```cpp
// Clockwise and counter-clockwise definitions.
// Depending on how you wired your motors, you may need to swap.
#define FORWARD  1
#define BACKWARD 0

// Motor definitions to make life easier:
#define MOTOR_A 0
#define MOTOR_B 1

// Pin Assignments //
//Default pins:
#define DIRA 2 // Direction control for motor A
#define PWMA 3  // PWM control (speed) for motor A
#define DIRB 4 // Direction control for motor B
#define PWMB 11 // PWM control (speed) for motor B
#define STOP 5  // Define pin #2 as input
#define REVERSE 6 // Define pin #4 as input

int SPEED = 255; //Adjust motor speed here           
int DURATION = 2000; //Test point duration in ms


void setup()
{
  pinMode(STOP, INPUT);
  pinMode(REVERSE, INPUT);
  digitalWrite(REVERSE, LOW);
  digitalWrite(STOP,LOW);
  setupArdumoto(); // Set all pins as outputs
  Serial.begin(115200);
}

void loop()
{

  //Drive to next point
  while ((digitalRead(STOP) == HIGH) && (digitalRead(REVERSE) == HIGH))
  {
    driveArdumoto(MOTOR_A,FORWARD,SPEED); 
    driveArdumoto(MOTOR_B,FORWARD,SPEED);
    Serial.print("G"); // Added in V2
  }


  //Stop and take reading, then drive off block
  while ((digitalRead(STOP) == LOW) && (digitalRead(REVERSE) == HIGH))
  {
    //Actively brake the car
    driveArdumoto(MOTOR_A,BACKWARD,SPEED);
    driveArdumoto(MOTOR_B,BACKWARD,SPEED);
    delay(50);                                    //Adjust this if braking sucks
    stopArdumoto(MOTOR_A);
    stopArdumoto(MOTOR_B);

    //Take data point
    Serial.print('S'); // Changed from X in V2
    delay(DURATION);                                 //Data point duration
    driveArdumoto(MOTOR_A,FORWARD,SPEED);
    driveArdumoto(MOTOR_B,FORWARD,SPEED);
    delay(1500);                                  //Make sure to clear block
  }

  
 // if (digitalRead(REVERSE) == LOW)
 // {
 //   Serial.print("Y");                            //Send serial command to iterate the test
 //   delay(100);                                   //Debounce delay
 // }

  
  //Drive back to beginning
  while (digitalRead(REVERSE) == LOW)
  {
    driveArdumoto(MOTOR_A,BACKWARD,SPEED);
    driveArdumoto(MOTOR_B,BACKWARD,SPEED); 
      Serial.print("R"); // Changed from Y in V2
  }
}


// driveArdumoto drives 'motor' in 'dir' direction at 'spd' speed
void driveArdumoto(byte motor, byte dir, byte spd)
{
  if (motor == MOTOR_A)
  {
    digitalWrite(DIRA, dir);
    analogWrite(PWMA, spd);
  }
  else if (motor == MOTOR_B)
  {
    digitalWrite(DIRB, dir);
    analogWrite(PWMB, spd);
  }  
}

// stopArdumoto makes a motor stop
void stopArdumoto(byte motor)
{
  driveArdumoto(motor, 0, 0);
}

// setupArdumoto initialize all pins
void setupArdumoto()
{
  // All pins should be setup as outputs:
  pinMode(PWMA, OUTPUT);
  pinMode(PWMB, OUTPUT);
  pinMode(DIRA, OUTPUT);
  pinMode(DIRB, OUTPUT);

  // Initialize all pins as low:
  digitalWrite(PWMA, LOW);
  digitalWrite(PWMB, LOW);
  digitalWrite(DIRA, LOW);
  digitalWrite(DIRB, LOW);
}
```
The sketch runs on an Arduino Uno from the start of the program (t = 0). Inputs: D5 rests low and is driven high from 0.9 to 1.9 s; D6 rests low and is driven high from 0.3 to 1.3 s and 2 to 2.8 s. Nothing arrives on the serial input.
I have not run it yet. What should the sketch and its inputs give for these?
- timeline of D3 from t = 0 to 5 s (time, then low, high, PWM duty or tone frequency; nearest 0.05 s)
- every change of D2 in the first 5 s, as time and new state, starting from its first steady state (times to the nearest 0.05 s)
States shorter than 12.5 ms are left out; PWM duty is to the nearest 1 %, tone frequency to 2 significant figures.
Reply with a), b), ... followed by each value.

a) 0 s high; 0.35 s low; 2.35 s high
b) 0 s low; 2.35 s high; 3.85 s low
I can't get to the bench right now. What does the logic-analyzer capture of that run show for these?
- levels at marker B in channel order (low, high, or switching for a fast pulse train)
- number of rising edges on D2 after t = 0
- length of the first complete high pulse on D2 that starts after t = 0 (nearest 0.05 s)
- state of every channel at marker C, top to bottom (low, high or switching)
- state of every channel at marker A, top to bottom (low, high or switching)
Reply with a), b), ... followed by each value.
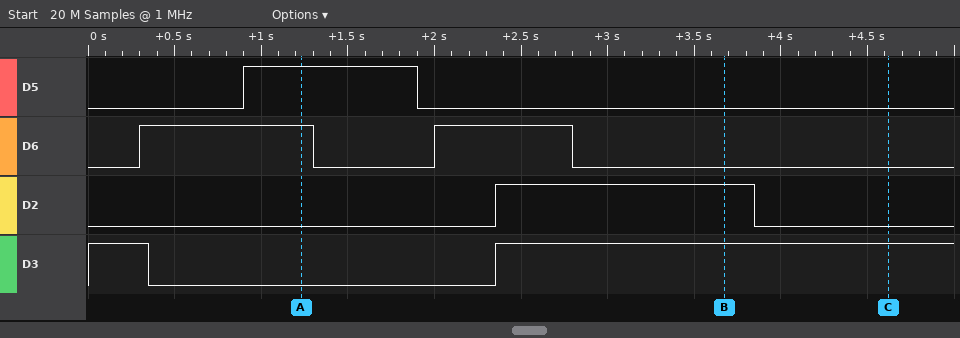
a) D5 low, D6 low, D2 high, D3 high
b) 1
c) 1.50 s
d) D5 low, D6 low, D2 low, D3 high
e) D5 high, D6 high, D2 low, D3 low
